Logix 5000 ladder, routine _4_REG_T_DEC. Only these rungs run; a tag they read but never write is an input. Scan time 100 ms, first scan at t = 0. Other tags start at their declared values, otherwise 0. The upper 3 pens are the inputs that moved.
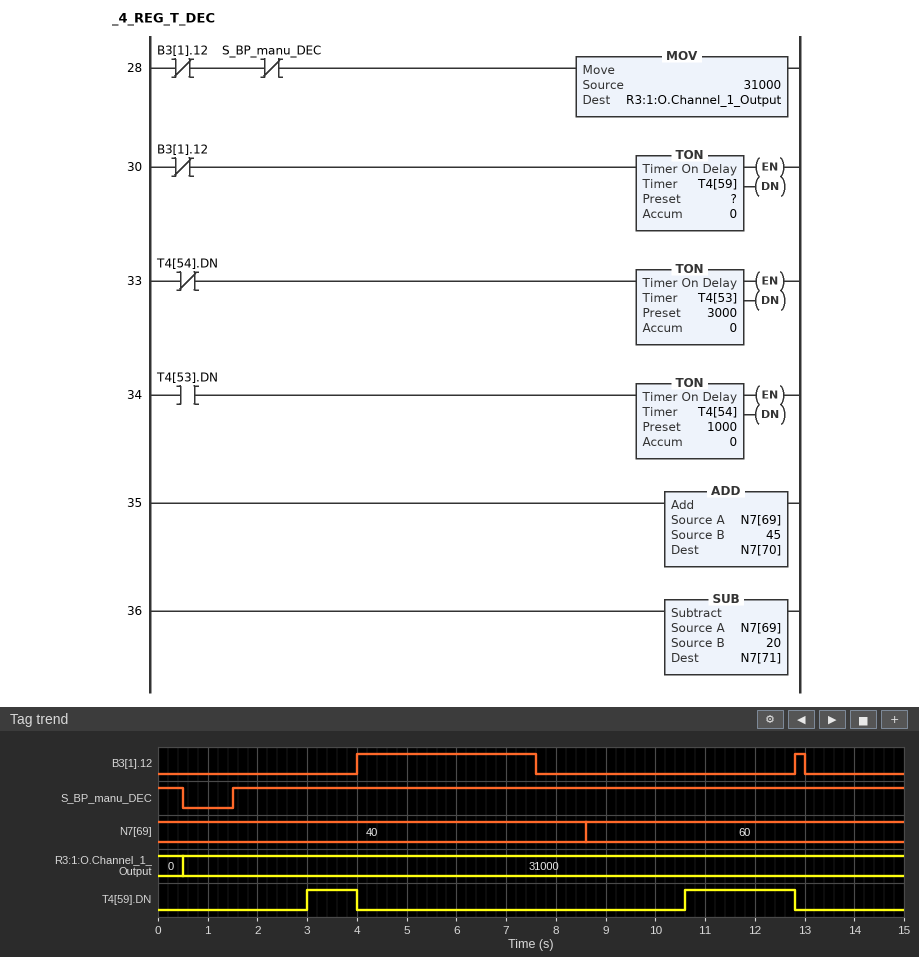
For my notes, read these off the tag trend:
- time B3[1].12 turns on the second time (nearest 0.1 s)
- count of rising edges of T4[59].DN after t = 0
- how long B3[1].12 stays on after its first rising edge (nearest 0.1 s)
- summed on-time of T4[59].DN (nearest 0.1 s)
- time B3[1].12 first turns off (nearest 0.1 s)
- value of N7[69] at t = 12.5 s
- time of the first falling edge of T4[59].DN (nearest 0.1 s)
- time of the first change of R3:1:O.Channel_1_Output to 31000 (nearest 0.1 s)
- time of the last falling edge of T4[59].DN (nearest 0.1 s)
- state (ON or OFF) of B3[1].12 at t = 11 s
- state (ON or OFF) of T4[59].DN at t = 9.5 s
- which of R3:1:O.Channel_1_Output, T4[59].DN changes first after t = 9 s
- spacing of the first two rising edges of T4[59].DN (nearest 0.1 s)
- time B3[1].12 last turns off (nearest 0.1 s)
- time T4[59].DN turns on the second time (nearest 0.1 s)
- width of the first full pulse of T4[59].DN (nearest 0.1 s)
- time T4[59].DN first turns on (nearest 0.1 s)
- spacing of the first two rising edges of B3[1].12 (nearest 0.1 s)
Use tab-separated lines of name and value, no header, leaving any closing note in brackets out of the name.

time B3[1].12 turns on the second time	12.8 s
count of rising edges of T4[59].DN after t = 0	2
how long B3[1].12 stays on after its first rising edge	3.6 s
summed on-time of T4[59].DN	3.2 s
time B3[1].12 first turns off	7.6 s
value of N7[69] at t = 12.5 s	60
time of the first falling edge of T4[59].DN	4.0 s
time of the first change of R3:1:O.Channel_1_Output to 31000	0.5 s
time of the last falling edge of T4[59].DN	12.8 s
state (ON or OFF) of B3[1].12 at t = 11 s	OFF
state (ON or OFF) of T4[59].DN at t = 9.5 s	OFF
which of R3:1:O.Channel_1_Output, T4[59].DN changes first after t = 9 s	T4[59].DN
spacing of the first two rising edges of T4[59].DN	7.6 s
time B3[1].12 last turns off	13.0 s
time T4[59].DN turns on the second time	10.6 s
width of the first full pulse of T4[59].DN	1.0 s
time T4[59].DN first turns on	3.0 s
spacing of the first two rising edges of B3[1].12	8.8 s
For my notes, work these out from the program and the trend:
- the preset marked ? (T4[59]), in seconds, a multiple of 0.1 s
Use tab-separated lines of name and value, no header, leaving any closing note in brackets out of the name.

the preset marked ? (T4[59]), in seconds, a multiple of 0.1 s	3.0 s
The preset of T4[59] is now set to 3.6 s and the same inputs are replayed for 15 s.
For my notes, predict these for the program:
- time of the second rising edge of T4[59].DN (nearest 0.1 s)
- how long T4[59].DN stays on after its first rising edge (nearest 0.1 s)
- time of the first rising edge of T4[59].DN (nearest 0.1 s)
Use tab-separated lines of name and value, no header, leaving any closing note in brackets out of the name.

time of the second rising edge of T4[59].DN	11.2 s
how long T4[59].DN stays on after its first rising edge	0.4 s
time of the first rising edge of T4[59].DN	3.6 s
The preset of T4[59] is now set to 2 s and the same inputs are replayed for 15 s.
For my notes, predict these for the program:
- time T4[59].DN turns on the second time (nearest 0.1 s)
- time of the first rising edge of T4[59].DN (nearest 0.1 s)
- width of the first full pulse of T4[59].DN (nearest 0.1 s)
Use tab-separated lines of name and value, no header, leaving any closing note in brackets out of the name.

time T4[59].DN turns on the second time	9.6 s
time of the first rising edge of T4[59].DN	2.0 s
width of the first full pulse of T4[59].DN	2.0 s
